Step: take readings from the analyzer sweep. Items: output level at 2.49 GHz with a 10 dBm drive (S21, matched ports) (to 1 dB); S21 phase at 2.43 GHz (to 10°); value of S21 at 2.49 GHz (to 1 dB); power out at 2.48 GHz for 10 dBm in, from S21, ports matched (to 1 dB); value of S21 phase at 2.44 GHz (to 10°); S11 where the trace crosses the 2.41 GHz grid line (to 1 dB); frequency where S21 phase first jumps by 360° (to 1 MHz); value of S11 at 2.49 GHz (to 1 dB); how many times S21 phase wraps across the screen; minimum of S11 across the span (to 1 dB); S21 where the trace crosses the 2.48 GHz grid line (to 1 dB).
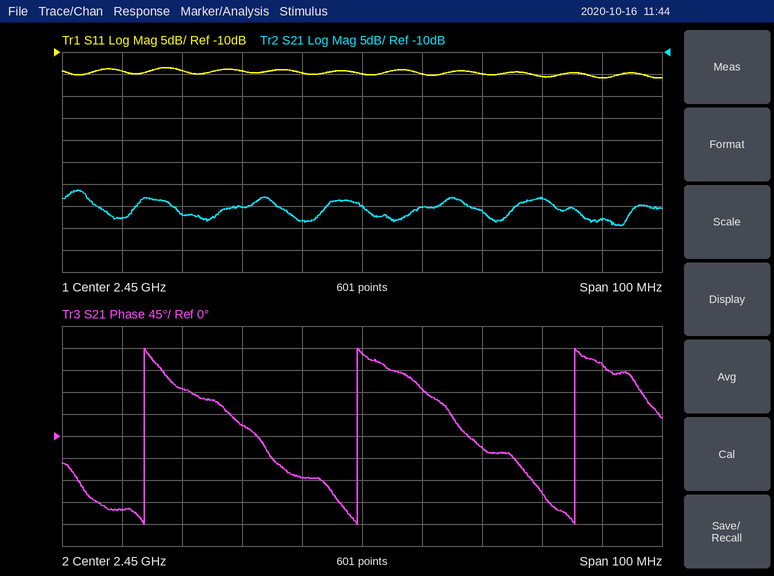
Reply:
-38 dBm
20°
-48 dB
-33 dBm
-80°
-14 dB
2.414 GHz
-16 dB
3
-16 dB
-43 dB
